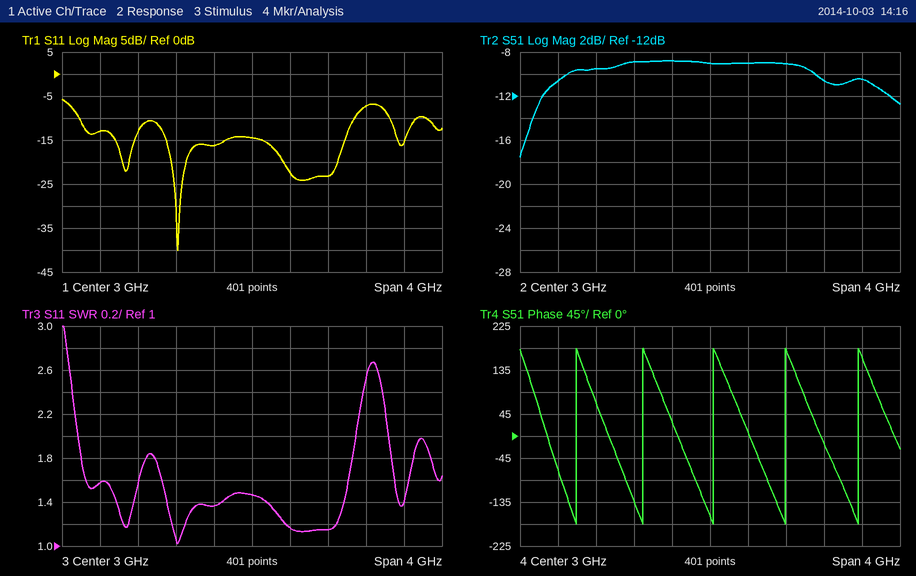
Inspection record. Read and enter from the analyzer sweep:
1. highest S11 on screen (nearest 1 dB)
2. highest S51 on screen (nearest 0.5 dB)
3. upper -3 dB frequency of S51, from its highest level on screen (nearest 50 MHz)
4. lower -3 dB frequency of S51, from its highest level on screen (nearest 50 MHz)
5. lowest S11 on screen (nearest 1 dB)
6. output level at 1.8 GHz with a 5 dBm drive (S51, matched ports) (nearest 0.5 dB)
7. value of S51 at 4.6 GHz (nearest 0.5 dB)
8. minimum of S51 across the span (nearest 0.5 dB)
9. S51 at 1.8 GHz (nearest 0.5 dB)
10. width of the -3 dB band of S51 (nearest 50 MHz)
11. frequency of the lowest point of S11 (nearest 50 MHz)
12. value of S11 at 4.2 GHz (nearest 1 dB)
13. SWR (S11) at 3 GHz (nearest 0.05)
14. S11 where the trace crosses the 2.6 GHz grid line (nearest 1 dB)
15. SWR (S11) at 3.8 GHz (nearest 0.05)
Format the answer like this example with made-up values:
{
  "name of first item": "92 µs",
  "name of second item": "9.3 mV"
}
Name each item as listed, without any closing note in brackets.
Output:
{
  "highest S11 on screen": "-6 dB",
  "highest S51 on screen": "-9.0 dB",
  "upper -3 dB frequency of S51, from its highest level on screen": "4.85 GHz",
  "lower -3 dB frequency of S51, from its highest level on screen": "1.25 GHz",
  "lowest S11 on screen": "-40 dB",
  "output level at 1.8 GHz with a 5 dBm drive (S51, matched ports)": "-4.5 dBm",
  "value of S51 at 4.6 GHz": "-10.5 dB",
  "minimum of S51 across the span": "-17.5 dB",
  "S51 at 1.8 GHz": "-9.5 dB",
  "width of the -3 dB band of S51": "3.60 GHz",
  "frequency of the lowest point of S11": "2.20 GHz",
  "value of S11 at 4.2 GHz": "-7 dB",
  "SWR (S11) at 3 GHz": "1.45",
  "S11 where the trace crosses the 2.6 GHz grid line": "-16 dB",
  "SWR (S11) at 3.8 GHz": "1.15"
}
